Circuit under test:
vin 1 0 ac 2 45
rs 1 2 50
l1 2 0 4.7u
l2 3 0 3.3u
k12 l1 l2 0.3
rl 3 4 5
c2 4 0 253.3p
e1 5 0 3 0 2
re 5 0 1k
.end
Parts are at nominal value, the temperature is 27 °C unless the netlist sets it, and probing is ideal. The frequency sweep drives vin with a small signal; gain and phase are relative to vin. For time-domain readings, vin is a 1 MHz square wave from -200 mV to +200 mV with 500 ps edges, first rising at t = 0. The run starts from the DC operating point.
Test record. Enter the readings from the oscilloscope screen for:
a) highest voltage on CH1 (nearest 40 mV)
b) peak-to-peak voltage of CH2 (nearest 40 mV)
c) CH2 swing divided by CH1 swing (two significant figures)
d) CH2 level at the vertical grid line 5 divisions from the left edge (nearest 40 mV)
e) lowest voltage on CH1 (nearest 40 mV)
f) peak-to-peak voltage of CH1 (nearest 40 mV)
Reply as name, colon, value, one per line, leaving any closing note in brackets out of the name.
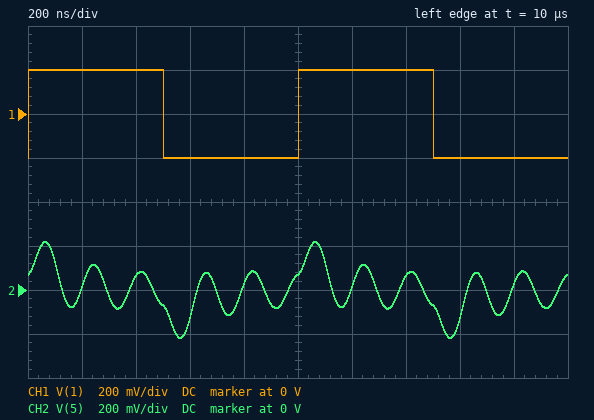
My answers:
highest voltage on CH1: 200 mV
peak-to-peak voltage of CH2: 440 mV
CH2 swing divided by CH1 swing: 1.1
CH2 level at the vertical grid line 5 divisions from the left edge: 80 mV
lowest voltage on CH1: -200 mV
peak-to-peak voltage of CH1: 400 mV
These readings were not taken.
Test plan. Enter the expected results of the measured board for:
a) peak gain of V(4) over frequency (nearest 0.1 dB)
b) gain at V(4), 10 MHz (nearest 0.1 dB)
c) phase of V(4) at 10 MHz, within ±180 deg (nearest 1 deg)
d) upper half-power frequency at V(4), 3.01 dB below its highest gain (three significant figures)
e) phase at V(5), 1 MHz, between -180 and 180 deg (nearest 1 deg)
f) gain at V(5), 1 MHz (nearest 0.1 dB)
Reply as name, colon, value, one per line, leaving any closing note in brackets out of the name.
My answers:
peak gain of V(4) over frequency: 10.5 dB
gain at V(4), 10 MHz: -18.2 dB
phase of V(4) at 10 MHz, within ±180 deg: -167 deg
upper half-power frequency at V(4), 3.01 dB below its highest gain: 5.95 MHz
phase at V(5), 1 MHz, between -180 and 180 deg: 59 deg
gain at V(5), 1 MHz: -11.6 dB
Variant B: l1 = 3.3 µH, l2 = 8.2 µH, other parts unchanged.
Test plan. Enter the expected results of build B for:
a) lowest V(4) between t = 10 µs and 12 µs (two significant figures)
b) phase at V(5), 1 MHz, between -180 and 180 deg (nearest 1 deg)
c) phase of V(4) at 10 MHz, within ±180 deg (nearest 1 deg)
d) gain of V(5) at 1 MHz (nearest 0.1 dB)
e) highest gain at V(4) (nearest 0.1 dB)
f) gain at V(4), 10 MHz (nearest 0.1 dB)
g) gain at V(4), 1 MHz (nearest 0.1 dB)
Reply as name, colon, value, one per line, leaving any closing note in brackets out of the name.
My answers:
lowest V(4) between t = 10 µs and 12 µs: -150 mV
phase at V(5), 1 MHz, between -180 and 180 deg: 67 deg
phase of V(4) at 10 MHz, within ±180 deg: -164 deg
gain of V(5) at 1 MHz: -8.1 dB
highest gain at V(4): 14.6 dB
gain at V(4), 10 MHz: -23.0 dB
gain at V(4), 1 MHz: -14.1 dB
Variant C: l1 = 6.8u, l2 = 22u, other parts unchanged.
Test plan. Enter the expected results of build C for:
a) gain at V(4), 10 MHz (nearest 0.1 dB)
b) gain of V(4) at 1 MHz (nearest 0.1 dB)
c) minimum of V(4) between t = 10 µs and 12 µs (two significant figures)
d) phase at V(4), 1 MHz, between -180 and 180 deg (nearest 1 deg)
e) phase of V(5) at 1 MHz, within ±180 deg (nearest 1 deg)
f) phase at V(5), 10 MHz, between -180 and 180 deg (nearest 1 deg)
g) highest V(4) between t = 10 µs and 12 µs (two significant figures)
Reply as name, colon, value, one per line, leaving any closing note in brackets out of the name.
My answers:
gain at V(4), 10 MHz: -31.0 dB
gain of V(4) at 1 MHz: -7.0 dB
minimum of V(4) between t = 10 µs and 12 µs: -140 mV
phase at V(4), 1 MHz, between -180 and 180 deg: 48 deg
phase of V(5) at 1 MHz, within ±180 deg: 49 deg
phase at V(5), 10 MHz, between -180 and 180 deg: -168 deg
highest V(4) between t = 10 µs and 12 µs: 140 mV
